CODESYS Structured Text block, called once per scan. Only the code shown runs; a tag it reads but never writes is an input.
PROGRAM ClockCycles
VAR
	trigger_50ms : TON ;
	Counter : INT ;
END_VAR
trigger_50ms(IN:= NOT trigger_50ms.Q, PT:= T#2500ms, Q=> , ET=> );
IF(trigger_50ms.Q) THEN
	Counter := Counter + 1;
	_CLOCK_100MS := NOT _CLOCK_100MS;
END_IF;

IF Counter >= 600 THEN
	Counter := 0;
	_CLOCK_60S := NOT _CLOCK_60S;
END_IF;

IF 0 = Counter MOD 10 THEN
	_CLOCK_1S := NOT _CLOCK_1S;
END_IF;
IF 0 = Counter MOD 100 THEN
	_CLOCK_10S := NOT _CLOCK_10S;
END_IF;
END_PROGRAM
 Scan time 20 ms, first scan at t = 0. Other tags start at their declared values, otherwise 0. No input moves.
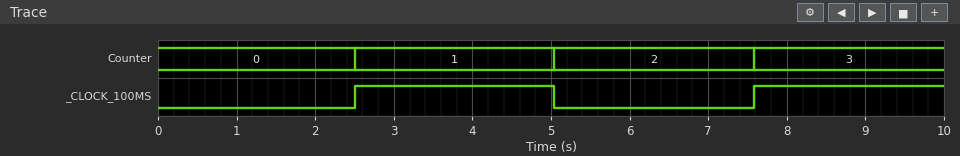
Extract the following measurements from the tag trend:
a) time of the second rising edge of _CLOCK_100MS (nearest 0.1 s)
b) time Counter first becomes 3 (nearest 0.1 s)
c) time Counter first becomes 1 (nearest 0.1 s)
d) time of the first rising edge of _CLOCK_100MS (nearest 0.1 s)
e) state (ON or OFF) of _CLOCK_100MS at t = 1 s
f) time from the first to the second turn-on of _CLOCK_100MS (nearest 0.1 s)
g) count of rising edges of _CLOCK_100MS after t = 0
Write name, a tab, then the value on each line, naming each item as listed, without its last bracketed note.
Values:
time of the second rising edge of _CLOCK_100MS	7.6 s
time Counter first becomes 3	7.6 s
time Counter first becomes 1	2.5 s
time of the first rising edge of _CLOCK_100MS	2.5 s
state (ON or OFF) of _CLOCK_100MS at t = 1 s	OFF
time from the first to the second turn-on of _CLOCK_100MS	5.1 s
count of rising edges of _CLOCK_100MS after t = 0	2
